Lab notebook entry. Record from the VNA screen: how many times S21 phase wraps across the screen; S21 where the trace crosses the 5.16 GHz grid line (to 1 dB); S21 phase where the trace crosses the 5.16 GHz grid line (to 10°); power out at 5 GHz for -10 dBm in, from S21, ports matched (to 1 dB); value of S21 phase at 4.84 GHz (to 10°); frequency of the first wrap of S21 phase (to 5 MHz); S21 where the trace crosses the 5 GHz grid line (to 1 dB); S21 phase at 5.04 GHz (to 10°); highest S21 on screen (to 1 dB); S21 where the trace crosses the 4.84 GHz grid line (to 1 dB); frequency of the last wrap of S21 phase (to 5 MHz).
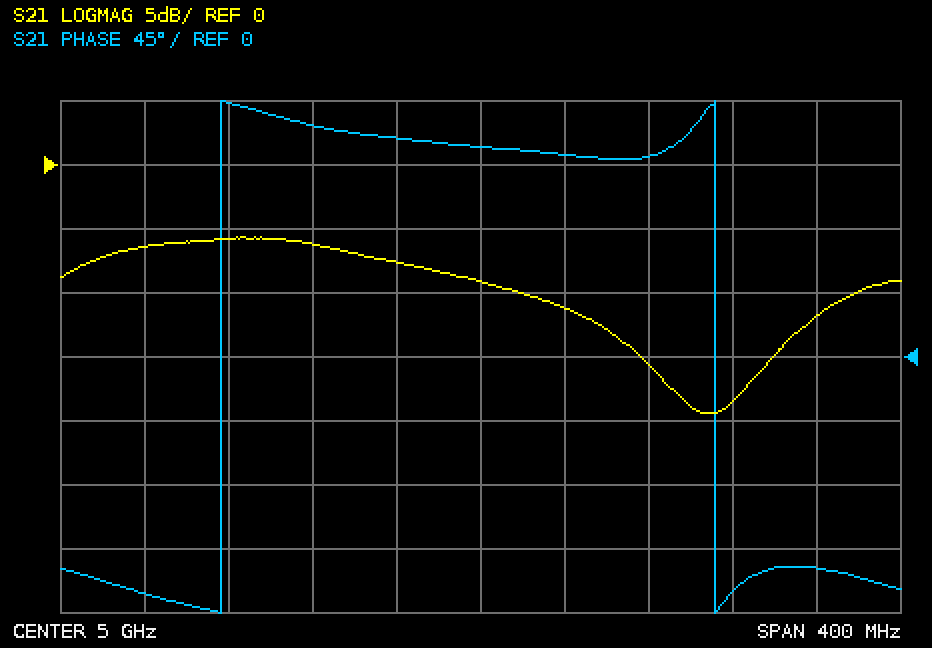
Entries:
2
-12 dB
-150°
-19 dBm
-170°
4.875 GHz
-9 dB
140°
-6 dB
-6 dB
5.110 GHz
